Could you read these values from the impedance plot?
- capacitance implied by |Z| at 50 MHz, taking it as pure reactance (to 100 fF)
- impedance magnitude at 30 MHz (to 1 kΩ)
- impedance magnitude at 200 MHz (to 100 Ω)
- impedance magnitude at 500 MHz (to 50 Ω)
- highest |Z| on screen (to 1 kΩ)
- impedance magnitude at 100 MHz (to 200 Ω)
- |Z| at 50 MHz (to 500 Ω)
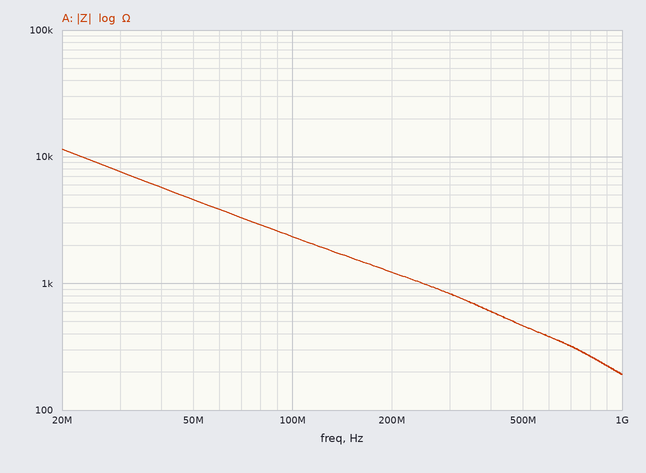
700 fF
8 kΩ
1.2 kΩ
450 Ω
11 kΩ
2.4 kΩ
4.5 kΩ
